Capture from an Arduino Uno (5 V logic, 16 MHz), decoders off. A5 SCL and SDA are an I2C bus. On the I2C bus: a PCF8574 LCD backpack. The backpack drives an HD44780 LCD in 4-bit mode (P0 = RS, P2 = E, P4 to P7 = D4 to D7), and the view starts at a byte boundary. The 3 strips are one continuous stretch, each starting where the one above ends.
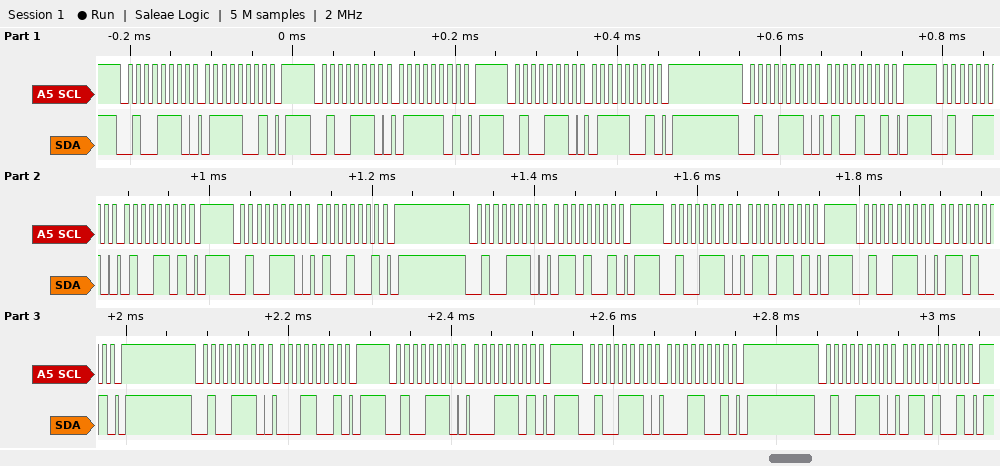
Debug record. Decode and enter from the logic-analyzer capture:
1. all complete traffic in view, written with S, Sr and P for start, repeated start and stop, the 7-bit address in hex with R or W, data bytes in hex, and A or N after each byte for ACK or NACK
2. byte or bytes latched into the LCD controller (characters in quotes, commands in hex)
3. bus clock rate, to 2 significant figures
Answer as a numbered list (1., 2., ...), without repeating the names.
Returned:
1. S 27W A 79 A P S 27W A 7D A P S 27W A 79 A P S 27W A 49 A P S 27W A 4D A P S 27W A 49 A P S 27W A 69 A P S 27W A 6D A P S 27W A 69 A P S 27W A 19 A P S 27W A 1D A P S 27W A 19 A P S 27W A 69 A P
2. 't' 'a'
3. 100 kHz
